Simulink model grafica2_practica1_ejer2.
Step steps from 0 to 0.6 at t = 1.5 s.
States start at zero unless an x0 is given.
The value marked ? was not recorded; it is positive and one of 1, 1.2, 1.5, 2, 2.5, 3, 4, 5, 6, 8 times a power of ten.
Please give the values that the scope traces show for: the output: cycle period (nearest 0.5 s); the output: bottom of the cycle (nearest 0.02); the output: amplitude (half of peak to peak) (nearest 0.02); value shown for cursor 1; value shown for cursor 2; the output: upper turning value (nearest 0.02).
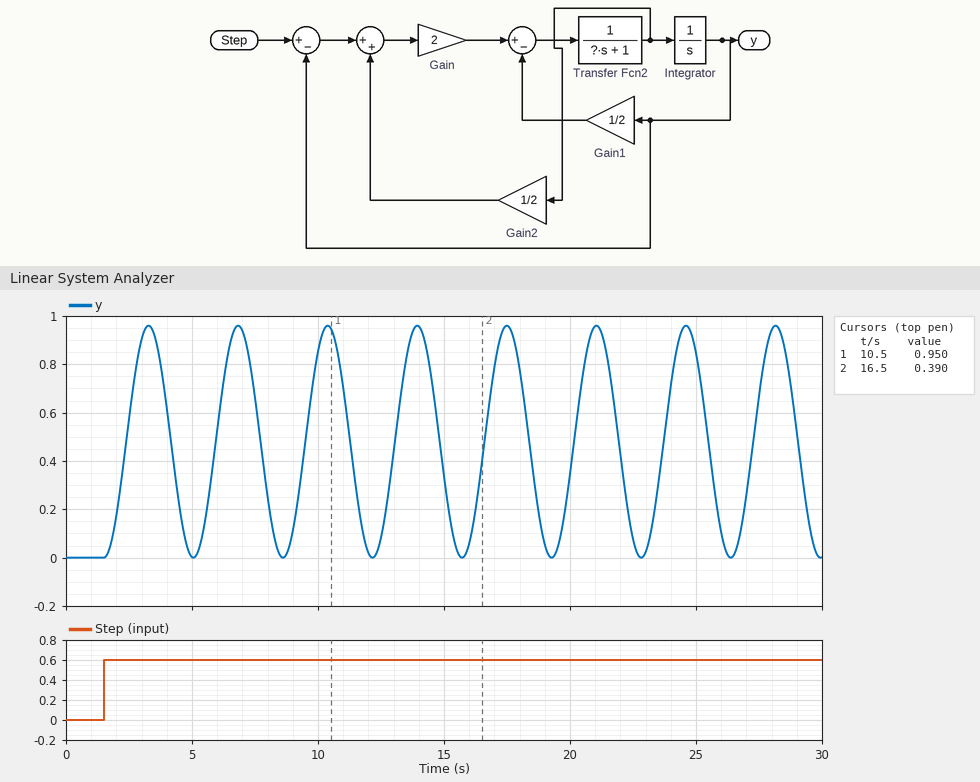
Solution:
3.5 s
0.00
0.48
0.950
0.390
0.96
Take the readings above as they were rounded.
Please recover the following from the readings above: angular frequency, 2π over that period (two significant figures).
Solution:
1.8 rad/s
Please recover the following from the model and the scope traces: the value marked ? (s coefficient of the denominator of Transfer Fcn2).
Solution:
0.8
